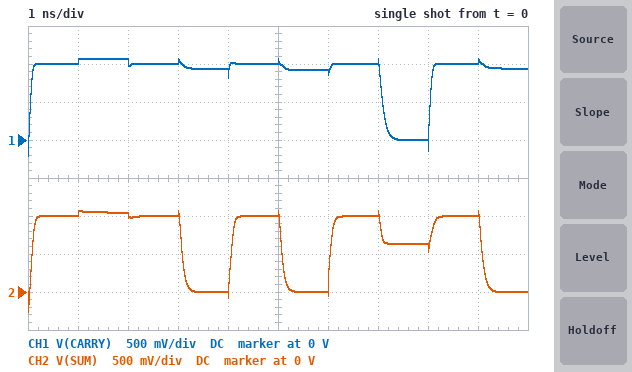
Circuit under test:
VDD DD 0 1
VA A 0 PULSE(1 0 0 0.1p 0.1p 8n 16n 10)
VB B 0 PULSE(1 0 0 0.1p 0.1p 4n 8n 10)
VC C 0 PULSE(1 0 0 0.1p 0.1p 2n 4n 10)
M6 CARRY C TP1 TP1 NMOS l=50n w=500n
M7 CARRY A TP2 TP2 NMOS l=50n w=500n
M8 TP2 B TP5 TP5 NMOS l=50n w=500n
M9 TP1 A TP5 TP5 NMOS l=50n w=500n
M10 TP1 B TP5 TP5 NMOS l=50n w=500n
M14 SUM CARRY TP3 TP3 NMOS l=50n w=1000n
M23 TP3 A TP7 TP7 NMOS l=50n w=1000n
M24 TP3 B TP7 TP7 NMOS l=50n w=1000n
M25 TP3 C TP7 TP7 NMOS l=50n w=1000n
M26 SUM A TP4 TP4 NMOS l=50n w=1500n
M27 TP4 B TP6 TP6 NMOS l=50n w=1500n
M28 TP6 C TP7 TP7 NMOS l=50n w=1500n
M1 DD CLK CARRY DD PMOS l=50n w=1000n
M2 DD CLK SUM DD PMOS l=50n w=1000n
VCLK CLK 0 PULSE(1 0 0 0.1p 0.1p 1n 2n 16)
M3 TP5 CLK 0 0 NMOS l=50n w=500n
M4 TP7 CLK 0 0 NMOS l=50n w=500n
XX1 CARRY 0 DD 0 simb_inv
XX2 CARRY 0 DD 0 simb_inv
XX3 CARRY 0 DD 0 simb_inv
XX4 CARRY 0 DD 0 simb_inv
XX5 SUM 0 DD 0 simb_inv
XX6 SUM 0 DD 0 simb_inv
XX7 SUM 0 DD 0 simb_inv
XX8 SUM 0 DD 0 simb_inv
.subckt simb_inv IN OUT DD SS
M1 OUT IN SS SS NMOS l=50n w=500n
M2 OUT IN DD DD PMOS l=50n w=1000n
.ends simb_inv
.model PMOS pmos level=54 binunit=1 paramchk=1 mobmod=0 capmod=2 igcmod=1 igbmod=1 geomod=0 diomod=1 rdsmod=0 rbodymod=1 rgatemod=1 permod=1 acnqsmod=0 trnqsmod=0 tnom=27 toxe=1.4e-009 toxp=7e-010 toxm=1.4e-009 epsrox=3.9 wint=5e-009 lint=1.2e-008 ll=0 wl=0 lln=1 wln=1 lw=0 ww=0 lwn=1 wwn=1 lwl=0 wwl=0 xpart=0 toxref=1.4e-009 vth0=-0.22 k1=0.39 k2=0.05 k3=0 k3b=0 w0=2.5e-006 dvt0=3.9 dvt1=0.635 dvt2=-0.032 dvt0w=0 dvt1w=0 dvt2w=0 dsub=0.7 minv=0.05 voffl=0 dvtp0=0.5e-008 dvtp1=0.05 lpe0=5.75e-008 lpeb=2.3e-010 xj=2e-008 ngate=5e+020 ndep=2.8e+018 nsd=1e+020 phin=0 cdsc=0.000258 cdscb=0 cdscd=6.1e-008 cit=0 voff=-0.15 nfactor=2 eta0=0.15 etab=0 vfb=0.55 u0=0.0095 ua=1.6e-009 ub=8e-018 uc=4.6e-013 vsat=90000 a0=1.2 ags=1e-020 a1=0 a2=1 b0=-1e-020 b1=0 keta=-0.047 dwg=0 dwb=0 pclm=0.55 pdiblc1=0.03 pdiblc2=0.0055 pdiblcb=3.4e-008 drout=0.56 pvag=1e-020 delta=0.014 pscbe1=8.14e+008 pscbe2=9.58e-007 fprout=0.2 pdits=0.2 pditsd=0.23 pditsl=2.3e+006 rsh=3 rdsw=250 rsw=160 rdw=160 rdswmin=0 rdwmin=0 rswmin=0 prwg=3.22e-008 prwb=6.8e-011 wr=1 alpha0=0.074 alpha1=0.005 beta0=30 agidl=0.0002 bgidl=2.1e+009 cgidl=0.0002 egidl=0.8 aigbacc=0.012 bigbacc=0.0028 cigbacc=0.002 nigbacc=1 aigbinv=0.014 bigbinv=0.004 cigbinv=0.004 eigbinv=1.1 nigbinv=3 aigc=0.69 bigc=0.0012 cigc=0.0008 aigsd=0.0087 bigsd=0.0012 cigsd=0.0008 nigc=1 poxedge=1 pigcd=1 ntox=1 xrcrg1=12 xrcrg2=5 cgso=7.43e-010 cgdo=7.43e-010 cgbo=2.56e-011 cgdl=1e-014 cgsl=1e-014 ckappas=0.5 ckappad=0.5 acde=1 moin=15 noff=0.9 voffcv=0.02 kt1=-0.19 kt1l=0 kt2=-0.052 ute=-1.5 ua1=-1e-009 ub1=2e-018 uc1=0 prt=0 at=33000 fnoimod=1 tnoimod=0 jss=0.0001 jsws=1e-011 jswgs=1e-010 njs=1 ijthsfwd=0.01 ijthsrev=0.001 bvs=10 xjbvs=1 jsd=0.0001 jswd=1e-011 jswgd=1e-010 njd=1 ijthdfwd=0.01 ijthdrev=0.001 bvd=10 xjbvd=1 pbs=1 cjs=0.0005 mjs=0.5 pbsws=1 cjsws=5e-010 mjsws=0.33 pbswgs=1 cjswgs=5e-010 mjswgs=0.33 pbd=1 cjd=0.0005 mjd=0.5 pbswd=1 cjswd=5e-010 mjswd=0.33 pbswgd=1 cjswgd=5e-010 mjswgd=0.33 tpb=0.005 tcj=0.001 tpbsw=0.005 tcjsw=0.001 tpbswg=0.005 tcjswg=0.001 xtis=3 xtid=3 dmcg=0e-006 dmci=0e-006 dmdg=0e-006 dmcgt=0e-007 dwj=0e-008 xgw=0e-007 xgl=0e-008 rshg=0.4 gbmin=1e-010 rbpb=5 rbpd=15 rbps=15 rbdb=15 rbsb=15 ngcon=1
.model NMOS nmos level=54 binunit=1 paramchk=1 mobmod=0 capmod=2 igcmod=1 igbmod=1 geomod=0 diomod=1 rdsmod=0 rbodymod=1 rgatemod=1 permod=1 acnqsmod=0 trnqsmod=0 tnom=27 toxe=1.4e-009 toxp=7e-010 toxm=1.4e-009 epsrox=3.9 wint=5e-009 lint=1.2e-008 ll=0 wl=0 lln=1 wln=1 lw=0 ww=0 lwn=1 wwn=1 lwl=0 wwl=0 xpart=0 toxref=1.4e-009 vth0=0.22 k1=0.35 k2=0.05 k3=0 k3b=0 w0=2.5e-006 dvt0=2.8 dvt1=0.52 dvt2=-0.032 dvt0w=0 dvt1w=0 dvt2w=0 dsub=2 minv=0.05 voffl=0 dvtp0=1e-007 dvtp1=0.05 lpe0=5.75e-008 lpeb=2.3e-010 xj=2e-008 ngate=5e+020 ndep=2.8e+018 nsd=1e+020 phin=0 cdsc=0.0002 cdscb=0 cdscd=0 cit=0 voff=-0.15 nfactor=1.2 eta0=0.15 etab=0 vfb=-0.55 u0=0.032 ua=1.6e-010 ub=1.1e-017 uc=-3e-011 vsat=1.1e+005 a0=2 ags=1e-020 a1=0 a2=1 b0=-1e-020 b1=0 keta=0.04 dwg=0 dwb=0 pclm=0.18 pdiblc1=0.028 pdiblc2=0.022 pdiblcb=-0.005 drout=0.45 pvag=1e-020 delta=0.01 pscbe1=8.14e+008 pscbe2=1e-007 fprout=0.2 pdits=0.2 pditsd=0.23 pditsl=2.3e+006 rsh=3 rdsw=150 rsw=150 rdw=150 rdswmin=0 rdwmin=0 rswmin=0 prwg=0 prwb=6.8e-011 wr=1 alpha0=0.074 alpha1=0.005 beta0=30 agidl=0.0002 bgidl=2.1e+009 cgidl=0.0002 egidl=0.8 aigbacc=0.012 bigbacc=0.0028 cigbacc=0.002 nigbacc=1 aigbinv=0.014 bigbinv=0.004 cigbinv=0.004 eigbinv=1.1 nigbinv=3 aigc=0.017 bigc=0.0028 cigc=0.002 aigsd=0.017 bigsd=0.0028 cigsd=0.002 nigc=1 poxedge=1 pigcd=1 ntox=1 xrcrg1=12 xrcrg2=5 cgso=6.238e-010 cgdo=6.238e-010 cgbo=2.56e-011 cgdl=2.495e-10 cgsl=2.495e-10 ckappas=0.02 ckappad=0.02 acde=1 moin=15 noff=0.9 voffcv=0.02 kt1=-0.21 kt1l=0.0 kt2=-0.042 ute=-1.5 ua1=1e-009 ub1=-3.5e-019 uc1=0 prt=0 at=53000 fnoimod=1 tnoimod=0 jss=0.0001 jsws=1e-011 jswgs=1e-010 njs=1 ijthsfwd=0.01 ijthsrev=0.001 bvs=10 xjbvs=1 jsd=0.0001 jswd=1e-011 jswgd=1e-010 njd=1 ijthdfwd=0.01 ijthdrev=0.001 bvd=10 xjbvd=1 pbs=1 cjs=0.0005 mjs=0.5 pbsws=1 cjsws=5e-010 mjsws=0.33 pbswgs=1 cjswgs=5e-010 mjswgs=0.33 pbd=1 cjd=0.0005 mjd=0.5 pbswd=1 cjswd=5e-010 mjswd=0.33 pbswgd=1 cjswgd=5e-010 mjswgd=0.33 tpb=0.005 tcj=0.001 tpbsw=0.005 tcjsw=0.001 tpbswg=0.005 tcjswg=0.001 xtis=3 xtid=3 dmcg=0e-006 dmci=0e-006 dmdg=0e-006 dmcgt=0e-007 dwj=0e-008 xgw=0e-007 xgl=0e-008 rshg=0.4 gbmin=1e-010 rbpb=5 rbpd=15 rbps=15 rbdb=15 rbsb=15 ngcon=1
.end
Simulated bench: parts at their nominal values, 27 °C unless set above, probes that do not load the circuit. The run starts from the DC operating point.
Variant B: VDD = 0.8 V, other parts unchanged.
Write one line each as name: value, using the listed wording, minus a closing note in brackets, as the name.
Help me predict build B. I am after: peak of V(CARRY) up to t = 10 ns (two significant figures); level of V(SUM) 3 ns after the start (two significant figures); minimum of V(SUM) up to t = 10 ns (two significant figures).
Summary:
peak of V(CARRY) up to t = 10 ns: 860 mV
level of V(SUM) 3 ns after the start: 800 mV
minimum of V(SUM) up to t = 10 ns: -300 mV
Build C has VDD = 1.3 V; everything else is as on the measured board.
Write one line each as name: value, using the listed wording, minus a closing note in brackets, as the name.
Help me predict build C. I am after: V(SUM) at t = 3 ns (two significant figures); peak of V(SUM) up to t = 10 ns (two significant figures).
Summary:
V(SUM) at t = 3 ns: 1.3 V
peak of V(SUM) up to t = 10 ns: 1.4 V
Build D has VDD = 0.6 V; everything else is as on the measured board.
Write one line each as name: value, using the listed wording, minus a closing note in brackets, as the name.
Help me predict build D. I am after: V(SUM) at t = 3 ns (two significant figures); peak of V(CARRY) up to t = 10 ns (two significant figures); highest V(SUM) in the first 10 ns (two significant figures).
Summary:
V(SUM) at t = 3 ns: 600 mV
peak of V(CARRY) up to t = 10 ns: 660 mV
highest V(SUM) in the first 10 ns: 650 mV
